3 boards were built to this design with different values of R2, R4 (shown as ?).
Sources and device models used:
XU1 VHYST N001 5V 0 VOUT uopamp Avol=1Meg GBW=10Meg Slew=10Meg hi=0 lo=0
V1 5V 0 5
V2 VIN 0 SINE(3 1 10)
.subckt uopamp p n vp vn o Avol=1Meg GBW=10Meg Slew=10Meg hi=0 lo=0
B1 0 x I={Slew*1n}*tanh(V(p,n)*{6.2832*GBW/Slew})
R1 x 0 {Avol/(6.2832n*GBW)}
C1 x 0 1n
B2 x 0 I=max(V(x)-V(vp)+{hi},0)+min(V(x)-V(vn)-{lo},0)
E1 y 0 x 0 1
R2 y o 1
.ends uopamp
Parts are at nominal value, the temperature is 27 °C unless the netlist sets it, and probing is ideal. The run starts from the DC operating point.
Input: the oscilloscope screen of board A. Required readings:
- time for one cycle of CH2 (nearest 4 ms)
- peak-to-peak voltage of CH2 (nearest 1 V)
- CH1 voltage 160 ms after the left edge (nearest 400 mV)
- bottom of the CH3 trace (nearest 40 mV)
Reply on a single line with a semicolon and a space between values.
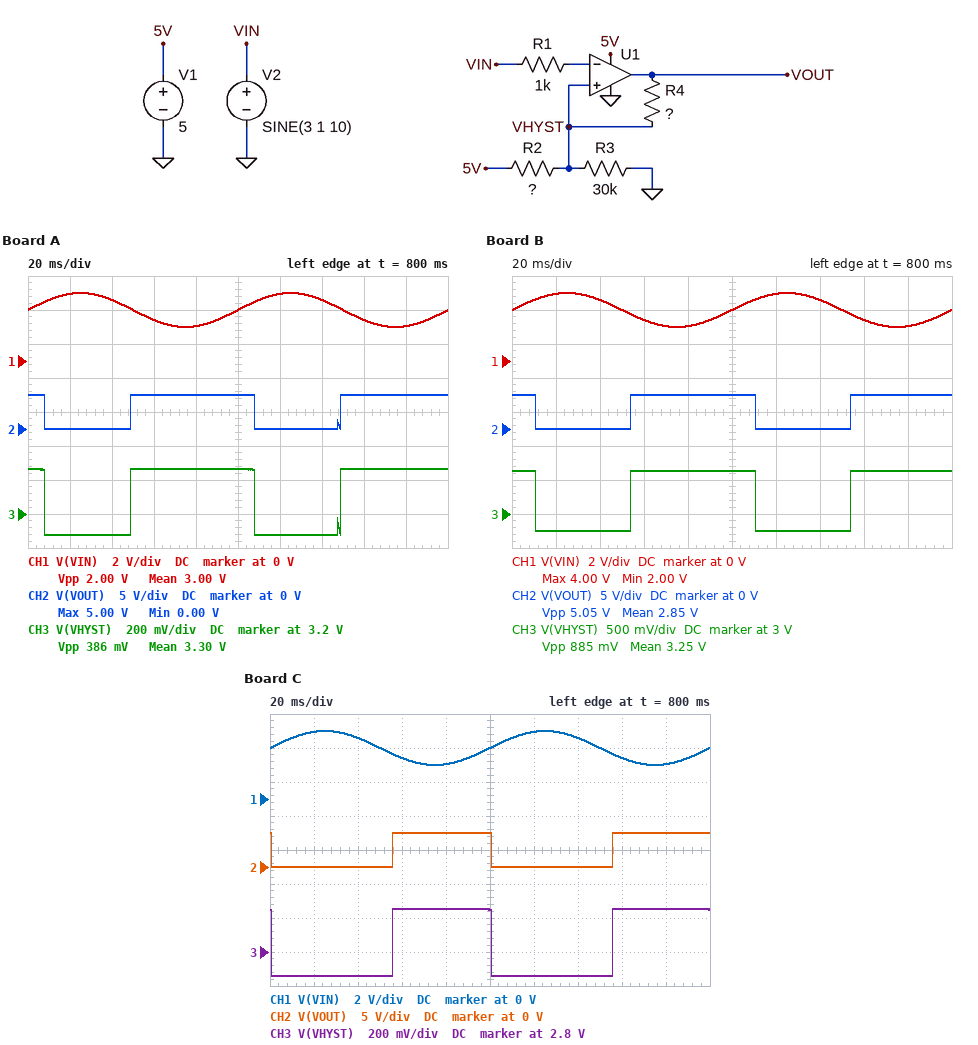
100 ms; 5 V; 2.4 V; 3.08 V
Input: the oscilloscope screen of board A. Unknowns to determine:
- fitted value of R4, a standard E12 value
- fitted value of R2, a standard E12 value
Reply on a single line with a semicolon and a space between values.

120 kΩ; 15 kΩ
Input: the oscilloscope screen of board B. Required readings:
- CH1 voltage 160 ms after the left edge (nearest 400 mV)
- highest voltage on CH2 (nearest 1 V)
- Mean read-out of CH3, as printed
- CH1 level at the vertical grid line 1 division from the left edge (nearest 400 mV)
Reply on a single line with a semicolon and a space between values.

2.4 V; 5 V; 3.25 V; 4.0 V
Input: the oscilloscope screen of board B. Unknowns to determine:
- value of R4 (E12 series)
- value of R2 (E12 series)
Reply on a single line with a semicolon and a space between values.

47 kΩ; 15 kΩ
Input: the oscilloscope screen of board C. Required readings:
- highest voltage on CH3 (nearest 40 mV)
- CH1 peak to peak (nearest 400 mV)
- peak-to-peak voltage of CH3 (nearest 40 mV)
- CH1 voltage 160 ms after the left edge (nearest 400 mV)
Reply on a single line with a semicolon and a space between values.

3.04 V; 2.0 V; 400 mV; 2.4 V
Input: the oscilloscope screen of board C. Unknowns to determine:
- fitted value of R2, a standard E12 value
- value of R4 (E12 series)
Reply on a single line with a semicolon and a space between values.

22 kΩ; 150 kΩ
